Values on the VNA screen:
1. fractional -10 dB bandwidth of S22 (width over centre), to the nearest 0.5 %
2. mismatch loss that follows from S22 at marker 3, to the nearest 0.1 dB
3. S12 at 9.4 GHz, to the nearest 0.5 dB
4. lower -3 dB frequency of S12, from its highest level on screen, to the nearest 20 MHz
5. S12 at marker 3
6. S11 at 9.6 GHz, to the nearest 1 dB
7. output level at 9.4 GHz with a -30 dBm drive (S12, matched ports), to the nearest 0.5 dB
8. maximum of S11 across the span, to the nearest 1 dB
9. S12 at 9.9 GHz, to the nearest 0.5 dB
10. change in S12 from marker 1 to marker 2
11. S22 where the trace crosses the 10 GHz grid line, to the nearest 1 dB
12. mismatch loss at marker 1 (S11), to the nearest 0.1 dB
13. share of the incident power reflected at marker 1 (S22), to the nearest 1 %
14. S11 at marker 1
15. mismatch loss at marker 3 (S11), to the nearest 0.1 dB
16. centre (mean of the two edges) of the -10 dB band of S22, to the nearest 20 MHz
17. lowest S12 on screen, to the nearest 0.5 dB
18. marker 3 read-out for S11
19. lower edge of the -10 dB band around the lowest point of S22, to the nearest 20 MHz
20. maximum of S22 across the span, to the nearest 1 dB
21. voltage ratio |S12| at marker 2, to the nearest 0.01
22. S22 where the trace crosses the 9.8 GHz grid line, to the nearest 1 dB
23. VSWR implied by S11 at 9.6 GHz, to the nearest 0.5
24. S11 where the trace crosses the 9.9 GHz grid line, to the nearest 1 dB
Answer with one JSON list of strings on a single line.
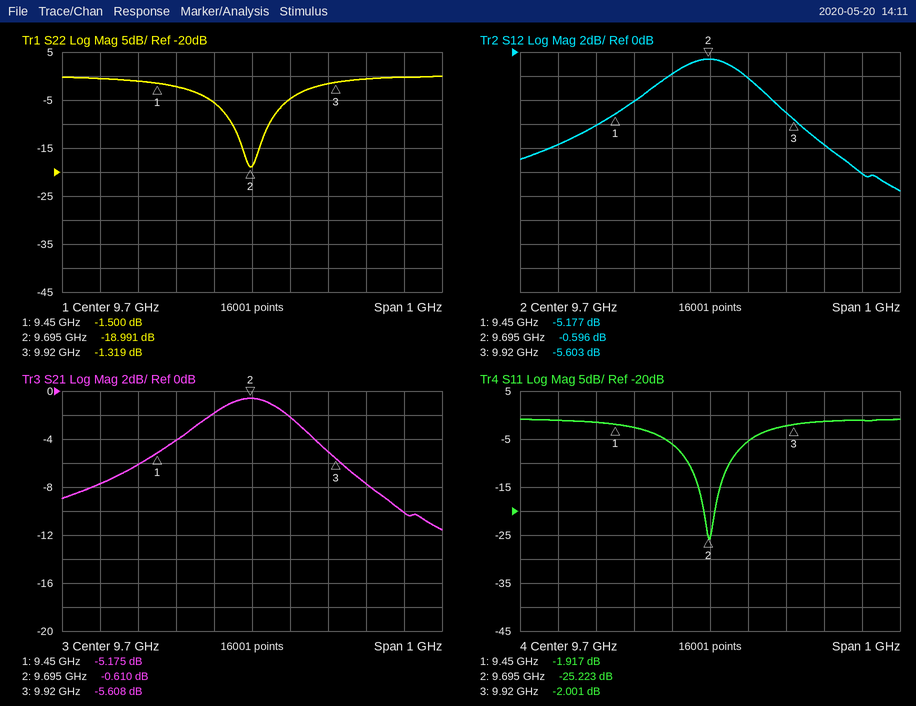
["1.0 %", "5.8 dB", "-6.0 dB", "9.52 GHz", "-5.603 dB", "-6 dB", "-36.0 dBm", "-1 dB", "-5.0 dB", "4.581 dB", "-1 dB", "4.5 dB", "71 %", "-1.917 dB", "4.3 dB", "9.70 GHz", "-11.5 dB", "-2.001 dB", "9.64 GHz", "0 dB", "0.93", "-5 dB", "3.0", "-2 dB"]
